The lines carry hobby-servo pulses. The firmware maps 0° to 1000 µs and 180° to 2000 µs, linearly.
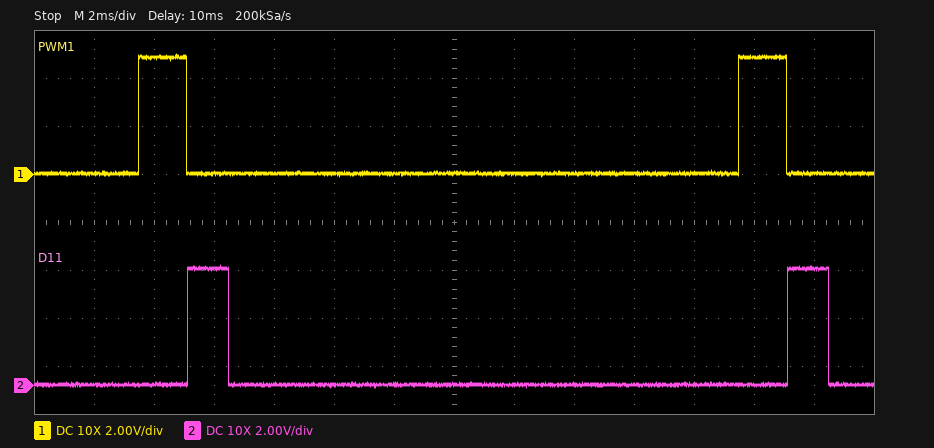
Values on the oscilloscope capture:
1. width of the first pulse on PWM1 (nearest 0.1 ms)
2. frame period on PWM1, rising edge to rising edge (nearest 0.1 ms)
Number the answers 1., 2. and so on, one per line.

1. 1.6 ms
2. 20.0 ms
